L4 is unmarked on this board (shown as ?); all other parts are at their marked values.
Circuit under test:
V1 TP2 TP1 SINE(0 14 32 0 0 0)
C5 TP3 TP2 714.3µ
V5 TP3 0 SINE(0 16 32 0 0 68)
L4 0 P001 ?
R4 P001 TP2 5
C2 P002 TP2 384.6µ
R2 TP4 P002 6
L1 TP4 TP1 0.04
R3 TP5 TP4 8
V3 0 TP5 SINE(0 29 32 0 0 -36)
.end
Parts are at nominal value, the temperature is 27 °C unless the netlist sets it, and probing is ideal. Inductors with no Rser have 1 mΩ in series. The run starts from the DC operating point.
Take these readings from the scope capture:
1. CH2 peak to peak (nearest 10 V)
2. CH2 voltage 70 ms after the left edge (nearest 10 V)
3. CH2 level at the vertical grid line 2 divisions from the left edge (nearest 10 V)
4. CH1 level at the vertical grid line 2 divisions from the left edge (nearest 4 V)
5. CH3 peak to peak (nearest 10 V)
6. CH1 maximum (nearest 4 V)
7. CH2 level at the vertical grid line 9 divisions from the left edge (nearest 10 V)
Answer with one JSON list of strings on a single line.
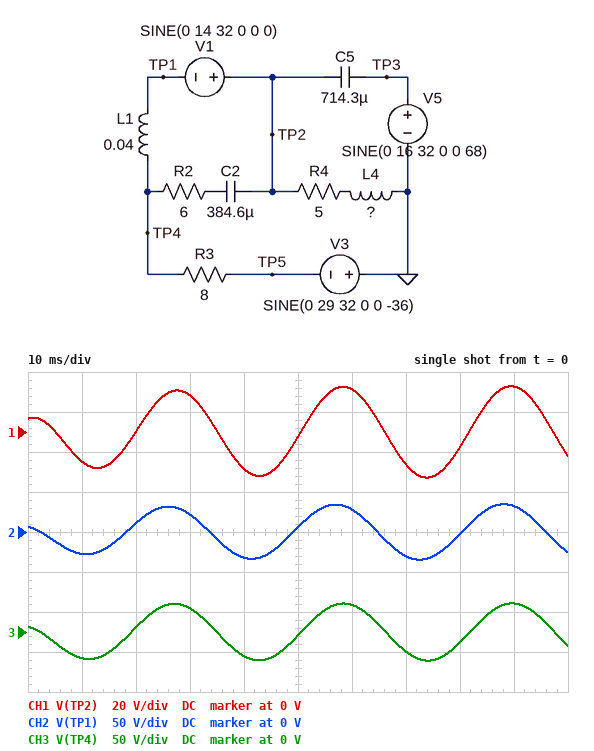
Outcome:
["70 V", "-30 V", "10 V", "0 V", "70 V", "24 V", "30 V"]
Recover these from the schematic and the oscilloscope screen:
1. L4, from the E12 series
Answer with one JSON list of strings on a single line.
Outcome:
["39 mH"]
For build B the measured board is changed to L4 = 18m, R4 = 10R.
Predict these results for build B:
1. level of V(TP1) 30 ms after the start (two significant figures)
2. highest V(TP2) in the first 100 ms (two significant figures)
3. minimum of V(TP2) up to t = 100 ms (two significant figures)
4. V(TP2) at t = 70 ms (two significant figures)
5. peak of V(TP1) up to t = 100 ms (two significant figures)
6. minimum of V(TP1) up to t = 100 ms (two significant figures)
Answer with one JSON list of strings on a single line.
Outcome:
["18 V", "15 V", "-15 V", "-6.5 V", "25 V", "-25 V"]
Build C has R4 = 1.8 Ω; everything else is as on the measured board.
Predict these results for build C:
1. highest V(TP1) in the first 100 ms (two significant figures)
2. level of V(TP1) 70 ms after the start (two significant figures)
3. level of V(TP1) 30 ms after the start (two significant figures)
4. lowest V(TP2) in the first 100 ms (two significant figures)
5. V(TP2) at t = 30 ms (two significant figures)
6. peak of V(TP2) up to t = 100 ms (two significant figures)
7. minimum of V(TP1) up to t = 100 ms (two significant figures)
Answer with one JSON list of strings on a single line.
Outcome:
["47 V", "-43 V", "23 V", "-33 V", "20 V", "33 V", "-46 V"]
